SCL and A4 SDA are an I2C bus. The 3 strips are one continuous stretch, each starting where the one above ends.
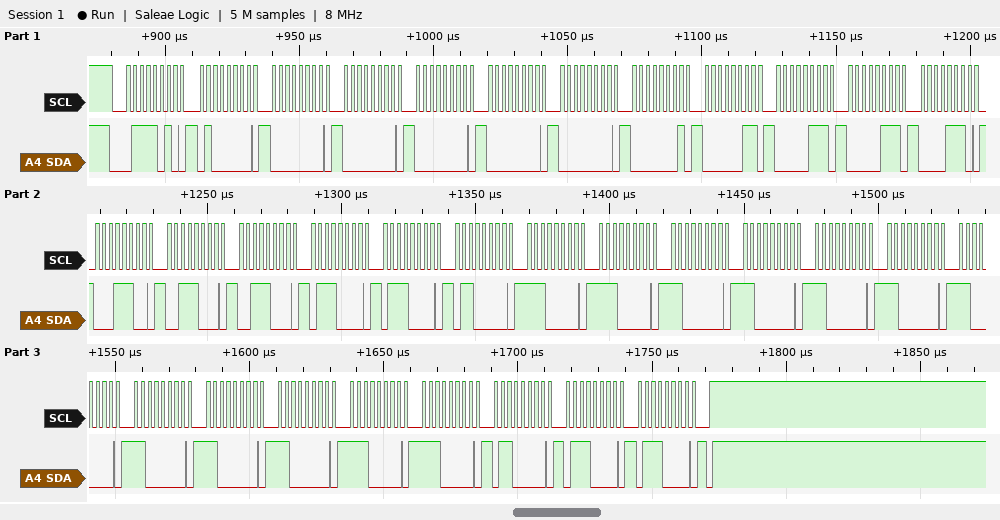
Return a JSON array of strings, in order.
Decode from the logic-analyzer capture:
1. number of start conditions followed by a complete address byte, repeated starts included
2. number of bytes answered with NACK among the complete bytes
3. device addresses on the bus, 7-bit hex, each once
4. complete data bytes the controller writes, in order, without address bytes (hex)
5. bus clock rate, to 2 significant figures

["1", "0", "0x3D", "40 00 00 00 00 00 01 03 07 07 0E 1C 38 38 70 70 60 E0 E0 C0 C0 C0 C0 C0 C0 C0 C0 E0 E0 60 70 70", "400 kHz"]
